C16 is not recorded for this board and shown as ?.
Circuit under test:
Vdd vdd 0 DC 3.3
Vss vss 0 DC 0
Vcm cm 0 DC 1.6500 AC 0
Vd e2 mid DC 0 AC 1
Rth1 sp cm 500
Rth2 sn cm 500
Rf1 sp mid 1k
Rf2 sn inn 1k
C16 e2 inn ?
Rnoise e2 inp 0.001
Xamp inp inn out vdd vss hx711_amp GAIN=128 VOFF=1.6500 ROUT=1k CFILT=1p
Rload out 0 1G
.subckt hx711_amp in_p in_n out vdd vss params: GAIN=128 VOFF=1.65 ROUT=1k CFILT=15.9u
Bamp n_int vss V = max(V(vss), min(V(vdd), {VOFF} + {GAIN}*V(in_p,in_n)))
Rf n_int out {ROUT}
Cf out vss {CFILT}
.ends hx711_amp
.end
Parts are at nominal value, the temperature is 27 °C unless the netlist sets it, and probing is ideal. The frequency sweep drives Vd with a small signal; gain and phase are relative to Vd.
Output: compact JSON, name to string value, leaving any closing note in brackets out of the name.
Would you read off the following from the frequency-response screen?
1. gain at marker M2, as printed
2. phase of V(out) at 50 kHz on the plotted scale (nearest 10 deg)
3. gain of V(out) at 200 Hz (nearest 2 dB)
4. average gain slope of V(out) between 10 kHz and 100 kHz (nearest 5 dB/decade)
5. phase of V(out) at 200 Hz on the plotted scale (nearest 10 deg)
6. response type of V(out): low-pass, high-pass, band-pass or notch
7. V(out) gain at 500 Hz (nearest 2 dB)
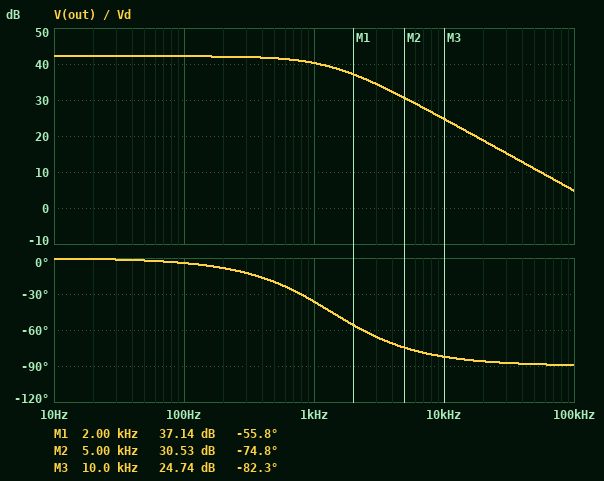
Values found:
{"gain at marker M2, as printed": "30.53 dB", "phase of V(out) at 50 kHz on the plotted scale": "-90 deg", "gain of V(out) at 200 Hz": "42 dB", "average gain slope of V(out) between 10 kHz and 100 kHz": "-20 dB/decade", "phase of V(out) at 200 Hz on the plotted scale": "-10 deg", "response type of V(out): low-pass, high-pass, band-pass or notch": "low-pass", "V(out) gain at 500 Hz": "42 dB"}
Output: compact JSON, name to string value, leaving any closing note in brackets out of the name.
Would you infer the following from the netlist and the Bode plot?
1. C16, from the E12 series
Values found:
{"C16, from the E12 series": "39 nF"}
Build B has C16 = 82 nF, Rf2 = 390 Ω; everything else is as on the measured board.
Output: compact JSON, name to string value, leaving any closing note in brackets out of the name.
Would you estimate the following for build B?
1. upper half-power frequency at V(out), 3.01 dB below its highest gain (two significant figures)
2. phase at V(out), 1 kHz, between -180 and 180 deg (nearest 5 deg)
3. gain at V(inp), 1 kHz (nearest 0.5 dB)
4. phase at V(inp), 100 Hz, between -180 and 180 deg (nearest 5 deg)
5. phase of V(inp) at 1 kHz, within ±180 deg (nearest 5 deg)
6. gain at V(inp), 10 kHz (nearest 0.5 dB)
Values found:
{"upper half-power frequency at V(out), 3.01 dB below its highest gain": "810 Hz", "phase at V(out), 1 kHz, between -180 and 180 deg": "-50 deg", "gain at V(inp), 1 kHz": "-3.0 dB", "phase at V(inp), 100 Hz, between -180 and 180 deg": "-5 deg", "phase of V(inp) at 1 kHz, within ±180 deg": "-25 deg", "gain at V(inp), 10 kHz": "-8.5 dB"}
